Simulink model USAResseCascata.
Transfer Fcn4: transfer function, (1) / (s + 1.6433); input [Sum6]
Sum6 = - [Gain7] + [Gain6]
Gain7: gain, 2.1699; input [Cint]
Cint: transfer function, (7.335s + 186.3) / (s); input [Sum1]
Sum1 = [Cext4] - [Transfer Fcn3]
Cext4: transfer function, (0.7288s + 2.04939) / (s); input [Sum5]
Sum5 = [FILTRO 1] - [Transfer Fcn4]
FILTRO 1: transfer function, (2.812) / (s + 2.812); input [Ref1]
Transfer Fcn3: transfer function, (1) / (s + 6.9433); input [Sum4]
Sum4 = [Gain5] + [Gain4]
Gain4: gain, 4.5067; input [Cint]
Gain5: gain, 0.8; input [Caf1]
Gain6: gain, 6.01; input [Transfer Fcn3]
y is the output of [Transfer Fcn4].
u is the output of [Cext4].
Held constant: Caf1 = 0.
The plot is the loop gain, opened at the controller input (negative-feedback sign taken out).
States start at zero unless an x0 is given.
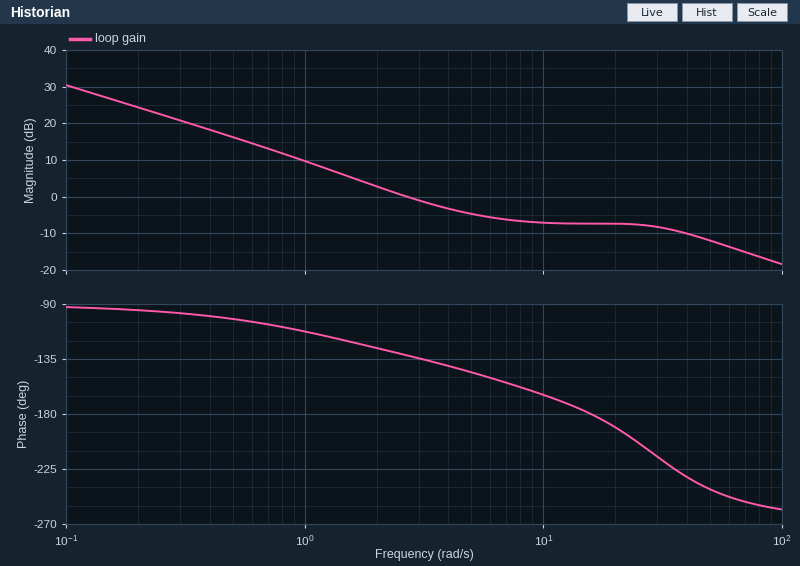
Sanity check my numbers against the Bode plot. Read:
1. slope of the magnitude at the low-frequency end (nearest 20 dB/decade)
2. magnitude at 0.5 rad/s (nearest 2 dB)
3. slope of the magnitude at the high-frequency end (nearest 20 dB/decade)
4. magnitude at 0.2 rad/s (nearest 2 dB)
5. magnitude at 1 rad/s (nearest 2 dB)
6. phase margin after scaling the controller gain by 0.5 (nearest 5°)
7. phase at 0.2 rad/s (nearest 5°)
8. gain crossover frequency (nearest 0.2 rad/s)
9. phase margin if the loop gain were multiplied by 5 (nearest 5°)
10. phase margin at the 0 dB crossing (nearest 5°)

-20 dB/decade
16 dB
-20 dB/decade
24 dB
10 dB
60°
-95°
2.6 rad/s
-70°
50°
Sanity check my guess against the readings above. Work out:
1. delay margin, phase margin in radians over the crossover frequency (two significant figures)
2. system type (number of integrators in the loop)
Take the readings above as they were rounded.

0.34 s
1
